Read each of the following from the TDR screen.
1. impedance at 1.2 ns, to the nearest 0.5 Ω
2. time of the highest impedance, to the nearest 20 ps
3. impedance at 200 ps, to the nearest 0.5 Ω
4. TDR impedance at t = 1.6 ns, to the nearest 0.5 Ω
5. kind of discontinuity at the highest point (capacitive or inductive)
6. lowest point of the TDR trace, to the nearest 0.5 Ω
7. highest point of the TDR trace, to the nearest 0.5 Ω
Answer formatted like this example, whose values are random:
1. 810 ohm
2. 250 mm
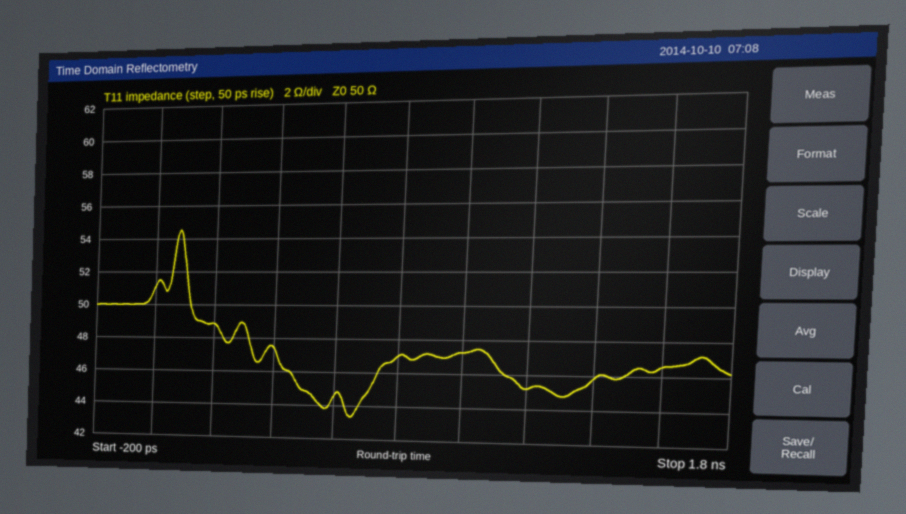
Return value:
1. 45.0 Ω
2. 80 ps
3. 49.0 Ω
4. 46.5 Ω
5. inductive
6. 43.5 Ω
7. 54.5 Ω
